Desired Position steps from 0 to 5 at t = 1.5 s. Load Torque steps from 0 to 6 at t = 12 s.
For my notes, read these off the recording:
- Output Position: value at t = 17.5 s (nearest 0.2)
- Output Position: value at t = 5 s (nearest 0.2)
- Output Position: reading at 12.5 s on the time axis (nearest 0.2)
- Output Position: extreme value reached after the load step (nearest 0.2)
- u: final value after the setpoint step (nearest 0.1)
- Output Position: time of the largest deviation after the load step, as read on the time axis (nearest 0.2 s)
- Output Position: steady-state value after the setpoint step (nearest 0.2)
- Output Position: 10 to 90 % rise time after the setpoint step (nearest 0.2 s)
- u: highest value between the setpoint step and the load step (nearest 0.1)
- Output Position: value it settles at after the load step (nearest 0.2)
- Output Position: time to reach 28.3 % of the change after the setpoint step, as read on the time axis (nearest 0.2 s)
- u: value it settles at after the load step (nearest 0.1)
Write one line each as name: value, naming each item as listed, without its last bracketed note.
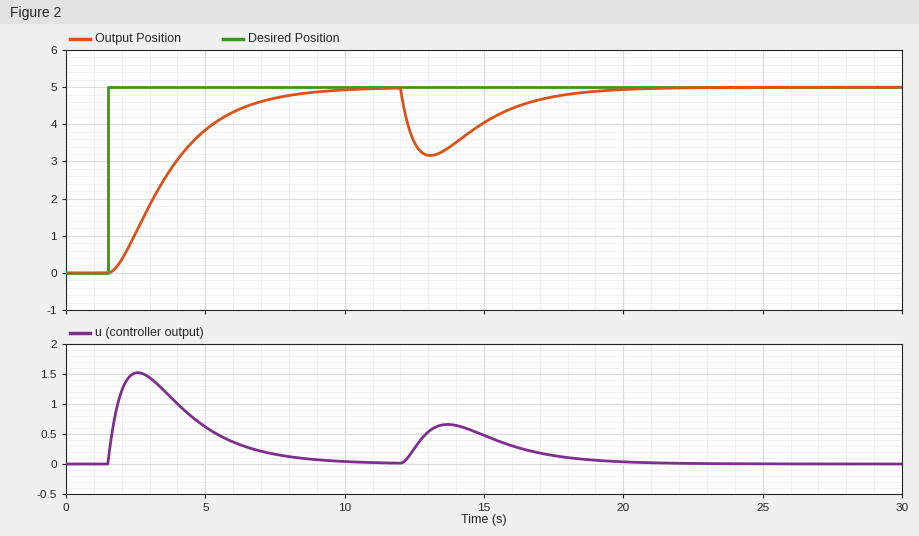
Output Position: value at t = 17.5 s: 4.8
Output Position: value at t = 5 s: 3.8
Output Position: reading at 12.5 s on the time axis: 3.6
Output Position: extreme value reached after the load step: 3.2
u: final value after the setpoint step: 0.0
Output Position: time of the largest deviation after the load step, as read on the time axis: 13.0 s
Output Position: steady-state value after the setpoint step: 5.0
Output Position: 10 to 90 % rise time after the setpoint step: 4.4 s
u: highest value between the setpoint step and the load step: 1.5
Output Position: value it settles at after the load step: 5.0
Output Position: time to reach 28.3 % of the change after the setpoint step, as read on the time axis: 2.8 s
u: value it settles at after the load step: 0.0
